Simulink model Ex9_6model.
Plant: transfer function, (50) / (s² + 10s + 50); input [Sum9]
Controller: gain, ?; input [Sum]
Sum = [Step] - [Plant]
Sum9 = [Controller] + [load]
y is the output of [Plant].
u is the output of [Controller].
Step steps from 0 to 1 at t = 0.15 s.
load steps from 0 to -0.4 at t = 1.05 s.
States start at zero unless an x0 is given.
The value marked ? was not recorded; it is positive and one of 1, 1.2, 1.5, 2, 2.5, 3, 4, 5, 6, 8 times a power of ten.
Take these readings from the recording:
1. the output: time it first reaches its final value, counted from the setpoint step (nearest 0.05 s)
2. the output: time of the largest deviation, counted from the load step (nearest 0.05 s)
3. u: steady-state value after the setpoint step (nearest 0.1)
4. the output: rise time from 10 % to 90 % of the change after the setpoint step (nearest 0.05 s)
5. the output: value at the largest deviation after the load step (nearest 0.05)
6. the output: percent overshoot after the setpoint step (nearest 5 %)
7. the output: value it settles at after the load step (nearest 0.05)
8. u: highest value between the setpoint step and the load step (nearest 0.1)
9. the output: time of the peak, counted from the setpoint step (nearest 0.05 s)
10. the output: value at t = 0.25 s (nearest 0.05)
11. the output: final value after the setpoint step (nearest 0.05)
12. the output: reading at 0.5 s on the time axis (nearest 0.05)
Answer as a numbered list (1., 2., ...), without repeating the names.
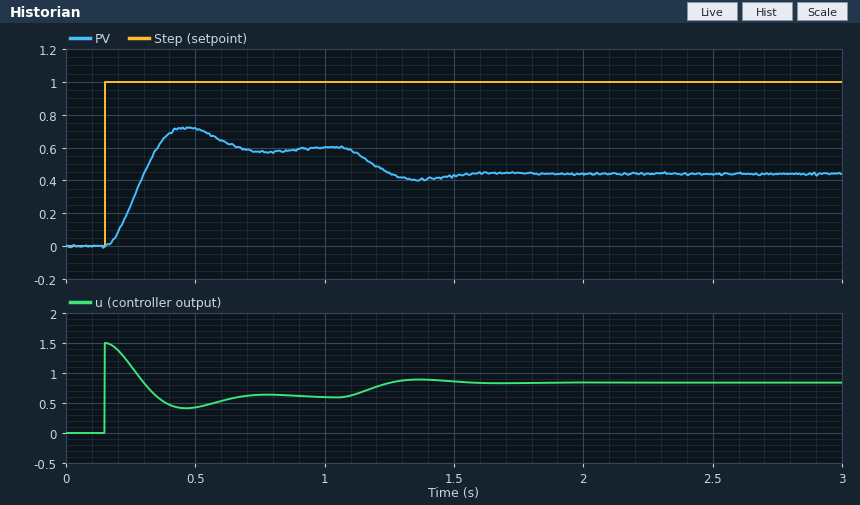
1. 0.20 s
2. 0.30 s
3. 0.6
4. 0.15 s
5. 0.40
6. 20 %
7. 0.45
8. 1.5
9. 0.30 s
10. 0.25
11. 0.60
12. 0.70
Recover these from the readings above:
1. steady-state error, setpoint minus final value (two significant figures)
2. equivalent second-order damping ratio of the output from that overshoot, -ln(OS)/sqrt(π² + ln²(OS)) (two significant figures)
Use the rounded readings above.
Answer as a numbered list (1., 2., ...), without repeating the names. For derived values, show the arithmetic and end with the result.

1. 1 - 0.6 = 0.40
2. ln(0.2) = -1.609; 1.609 / sqrt(9.870 + 2.590) = 0.46
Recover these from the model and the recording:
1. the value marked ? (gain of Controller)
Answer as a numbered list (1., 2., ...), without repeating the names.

1. 1.5
